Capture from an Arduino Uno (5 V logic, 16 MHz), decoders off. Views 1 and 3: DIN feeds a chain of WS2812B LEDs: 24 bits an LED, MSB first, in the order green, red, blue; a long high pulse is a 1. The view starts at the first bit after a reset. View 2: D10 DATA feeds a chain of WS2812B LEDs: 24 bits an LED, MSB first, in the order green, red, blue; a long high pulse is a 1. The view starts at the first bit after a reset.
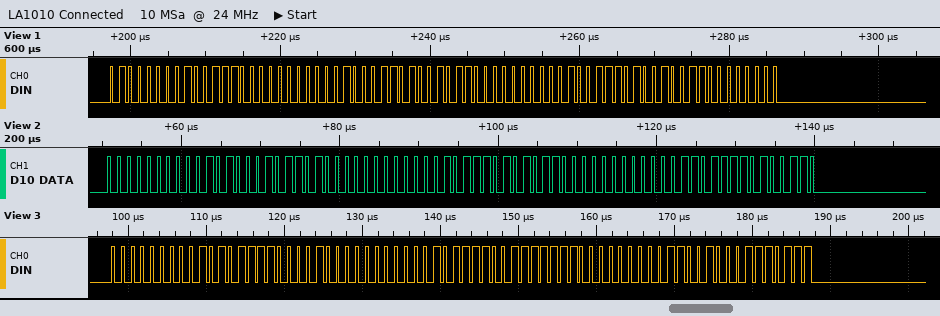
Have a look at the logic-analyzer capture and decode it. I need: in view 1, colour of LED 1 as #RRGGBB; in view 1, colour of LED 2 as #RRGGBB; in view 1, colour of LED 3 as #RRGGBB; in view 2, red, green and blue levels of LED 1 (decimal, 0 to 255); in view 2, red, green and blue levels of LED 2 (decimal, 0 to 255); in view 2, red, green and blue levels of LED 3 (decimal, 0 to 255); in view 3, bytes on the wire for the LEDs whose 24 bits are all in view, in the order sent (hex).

#9C4000
#964600
#934E00
40, 0, 180
46, 0, 172
55, 0, 166
00 57 84 00 5E 7F 00 64 77
